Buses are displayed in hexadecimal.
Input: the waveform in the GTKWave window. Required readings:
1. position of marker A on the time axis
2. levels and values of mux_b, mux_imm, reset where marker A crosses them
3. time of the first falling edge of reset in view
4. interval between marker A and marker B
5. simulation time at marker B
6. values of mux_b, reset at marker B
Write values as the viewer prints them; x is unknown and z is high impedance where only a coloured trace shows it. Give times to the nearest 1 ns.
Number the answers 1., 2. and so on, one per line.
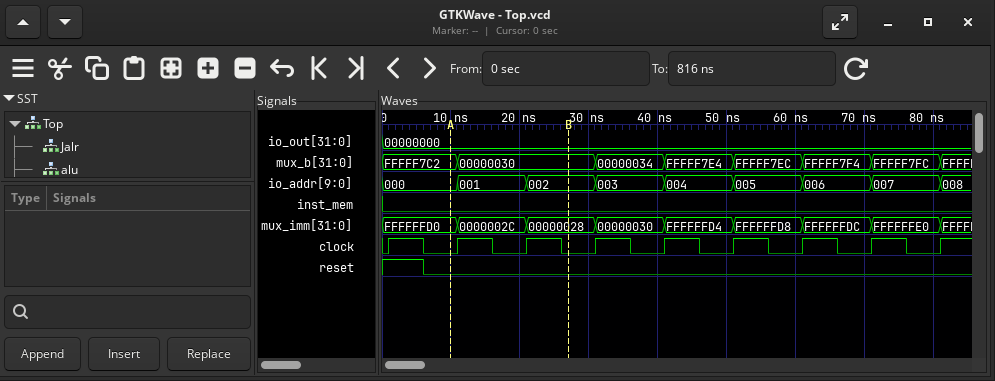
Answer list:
1. 10 ns
2. mux_b=FFFFF7C2, mux_imm=FFFFFFD0, reset=0
3. 6 ns
4. 17 ns
5. 27 ns
6. mux_b=00000030, reset=0
